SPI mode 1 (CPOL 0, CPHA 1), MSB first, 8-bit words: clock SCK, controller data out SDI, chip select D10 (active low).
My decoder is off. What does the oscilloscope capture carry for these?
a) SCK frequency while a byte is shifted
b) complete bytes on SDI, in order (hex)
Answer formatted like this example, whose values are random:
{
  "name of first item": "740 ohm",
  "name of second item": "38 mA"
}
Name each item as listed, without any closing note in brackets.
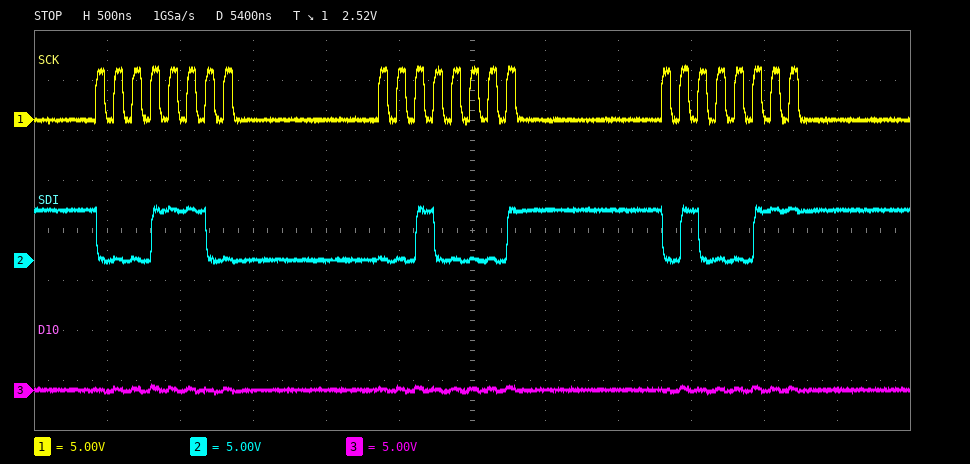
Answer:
{
  "SCK frequency while a byte is shifted": "8 MHz",
  "complete bytes on SDI, in order": "0x1C 0x21 0x47"
}
